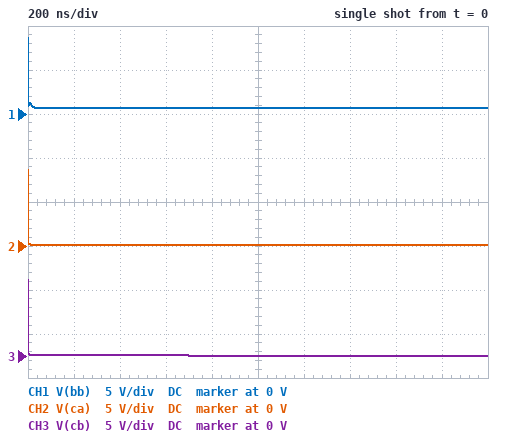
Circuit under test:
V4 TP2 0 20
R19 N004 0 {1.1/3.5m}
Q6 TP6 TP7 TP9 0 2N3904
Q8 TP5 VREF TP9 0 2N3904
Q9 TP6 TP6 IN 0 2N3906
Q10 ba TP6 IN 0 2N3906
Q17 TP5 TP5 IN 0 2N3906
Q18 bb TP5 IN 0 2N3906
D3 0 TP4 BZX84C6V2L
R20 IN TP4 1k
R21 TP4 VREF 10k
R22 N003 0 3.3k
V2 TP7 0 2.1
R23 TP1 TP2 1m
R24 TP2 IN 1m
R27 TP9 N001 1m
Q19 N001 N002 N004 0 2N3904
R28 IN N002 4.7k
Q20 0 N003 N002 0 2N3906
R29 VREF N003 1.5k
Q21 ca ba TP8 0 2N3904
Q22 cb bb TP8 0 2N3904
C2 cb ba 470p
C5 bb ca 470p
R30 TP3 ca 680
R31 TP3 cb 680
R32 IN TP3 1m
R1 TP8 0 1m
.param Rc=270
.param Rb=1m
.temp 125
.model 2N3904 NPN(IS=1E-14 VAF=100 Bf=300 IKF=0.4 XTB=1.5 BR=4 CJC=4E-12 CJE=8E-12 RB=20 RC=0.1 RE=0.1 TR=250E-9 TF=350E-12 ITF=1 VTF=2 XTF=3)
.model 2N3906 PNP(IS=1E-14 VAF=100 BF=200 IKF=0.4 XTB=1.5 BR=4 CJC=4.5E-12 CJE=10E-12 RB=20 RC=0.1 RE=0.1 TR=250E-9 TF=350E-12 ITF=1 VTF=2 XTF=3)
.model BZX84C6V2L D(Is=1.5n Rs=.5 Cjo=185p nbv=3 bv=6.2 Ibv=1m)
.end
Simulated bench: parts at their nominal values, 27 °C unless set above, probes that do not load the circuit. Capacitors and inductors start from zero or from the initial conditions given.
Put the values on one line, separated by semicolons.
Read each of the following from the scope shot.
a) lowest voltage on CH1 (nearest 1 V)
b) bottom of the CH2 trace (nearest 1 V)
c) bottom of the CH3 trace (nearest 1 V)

1 V; 0 V; 0 V
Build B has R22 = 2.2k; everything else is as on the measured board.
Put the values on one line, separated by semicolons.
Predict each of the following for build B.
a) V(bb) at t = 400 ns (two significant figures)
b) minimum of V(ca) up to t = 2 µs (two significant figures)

600 mV; 45 mV
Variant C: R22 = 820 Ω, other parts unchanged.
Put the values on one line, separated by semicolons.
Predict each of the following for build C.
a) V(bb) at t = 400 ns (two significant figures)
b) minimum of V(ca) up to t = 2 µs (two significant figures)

600 mV; 63 mV
